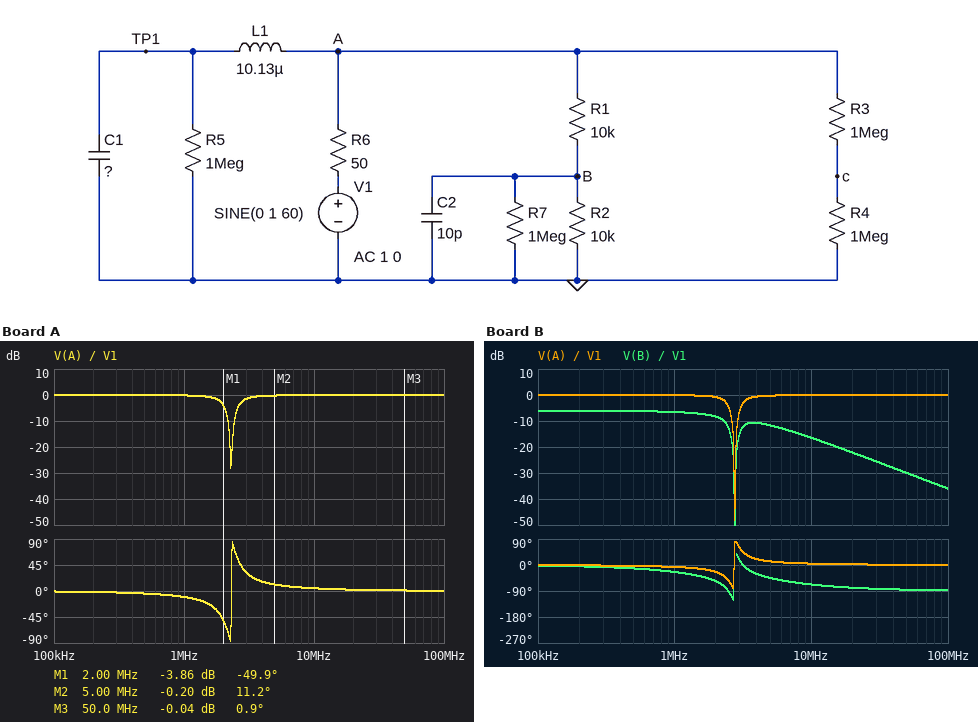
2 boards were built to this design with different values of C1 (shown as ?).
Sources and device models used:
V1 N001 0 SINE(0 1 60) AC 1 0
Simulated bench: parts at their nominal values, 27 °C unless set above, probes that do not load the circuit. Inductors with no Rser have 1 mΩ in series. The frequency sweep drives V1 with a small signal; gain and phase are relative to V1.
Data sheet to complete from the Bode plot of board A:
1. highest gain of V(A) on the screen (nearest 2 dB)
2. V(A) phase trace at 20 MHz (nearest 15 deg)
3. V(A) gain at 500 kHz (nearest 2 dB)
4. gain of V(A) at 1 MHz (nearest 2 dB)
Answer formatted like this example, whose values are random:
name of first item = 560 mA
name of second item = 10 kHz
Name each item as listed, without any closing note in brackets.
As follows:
highest gain of V(A) on the screen = 0 dB
V(A) phase trace at 20 MHz = 0 deg
V(A) gain at 500 kHz = 0 dB
gain of V(A) at 1 MHz = 0 dB
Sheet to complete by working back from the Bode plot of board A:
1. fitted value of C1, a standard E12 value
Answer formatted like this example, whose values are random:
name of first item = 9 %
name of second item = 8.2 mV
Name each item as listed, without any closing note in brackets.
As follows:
fitted value of C1, a standard E12 value = 470 pF
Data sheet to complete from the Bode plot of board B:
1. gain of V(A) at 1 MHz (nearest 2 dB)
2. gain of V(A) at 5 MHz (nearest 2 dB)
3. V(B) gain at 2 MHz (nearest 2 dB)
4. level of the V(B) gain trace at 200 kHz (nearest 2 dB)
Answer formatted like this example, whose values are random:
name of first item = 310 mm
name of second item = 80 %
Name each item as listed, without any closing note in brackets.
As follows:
gain of V(A) at 1 MHz = 0 dB
gain of V(A) at 5 MHz = 0 dB
V(B) gain at 2 MHz = -8 dB
level of the V(B) gain trace at 200 kHz = -6 dB
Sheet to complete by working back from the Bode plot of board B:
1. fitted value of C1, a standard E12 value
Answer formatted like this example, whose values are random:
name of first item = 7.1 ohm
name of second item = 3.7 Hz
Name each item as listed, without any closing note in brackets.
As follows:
fitted value of C1, a standard E12 value = 330 pF
